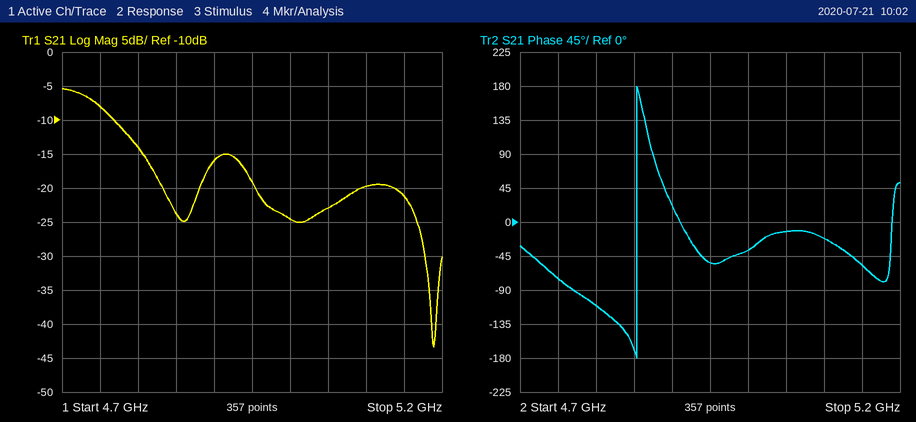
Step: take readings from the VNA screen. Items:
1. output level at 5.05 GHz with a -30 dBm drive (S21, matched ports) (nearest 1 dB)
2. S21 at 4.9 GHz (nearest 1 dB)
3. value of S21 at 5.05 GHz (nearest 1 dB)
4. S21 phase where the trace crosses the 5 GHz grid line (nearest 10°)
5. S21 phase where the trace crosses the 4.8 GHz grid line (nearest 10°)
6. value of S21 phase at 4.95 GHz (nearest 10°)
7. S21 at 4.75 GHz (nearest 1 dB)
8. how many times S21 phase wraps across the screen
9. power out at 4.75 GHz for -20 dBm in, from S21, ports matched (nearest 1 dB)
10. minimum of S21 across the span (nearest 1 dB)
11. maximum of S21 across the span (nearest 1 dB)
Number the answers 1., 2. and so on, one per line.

1. -53 dBm
2. -16 dB
3. -23 dB
4. -40°
5. -110°
6. -50°
7. -8 dB
8. 1
9. -28 dBm
10. -43 dB
11. -5 dB
